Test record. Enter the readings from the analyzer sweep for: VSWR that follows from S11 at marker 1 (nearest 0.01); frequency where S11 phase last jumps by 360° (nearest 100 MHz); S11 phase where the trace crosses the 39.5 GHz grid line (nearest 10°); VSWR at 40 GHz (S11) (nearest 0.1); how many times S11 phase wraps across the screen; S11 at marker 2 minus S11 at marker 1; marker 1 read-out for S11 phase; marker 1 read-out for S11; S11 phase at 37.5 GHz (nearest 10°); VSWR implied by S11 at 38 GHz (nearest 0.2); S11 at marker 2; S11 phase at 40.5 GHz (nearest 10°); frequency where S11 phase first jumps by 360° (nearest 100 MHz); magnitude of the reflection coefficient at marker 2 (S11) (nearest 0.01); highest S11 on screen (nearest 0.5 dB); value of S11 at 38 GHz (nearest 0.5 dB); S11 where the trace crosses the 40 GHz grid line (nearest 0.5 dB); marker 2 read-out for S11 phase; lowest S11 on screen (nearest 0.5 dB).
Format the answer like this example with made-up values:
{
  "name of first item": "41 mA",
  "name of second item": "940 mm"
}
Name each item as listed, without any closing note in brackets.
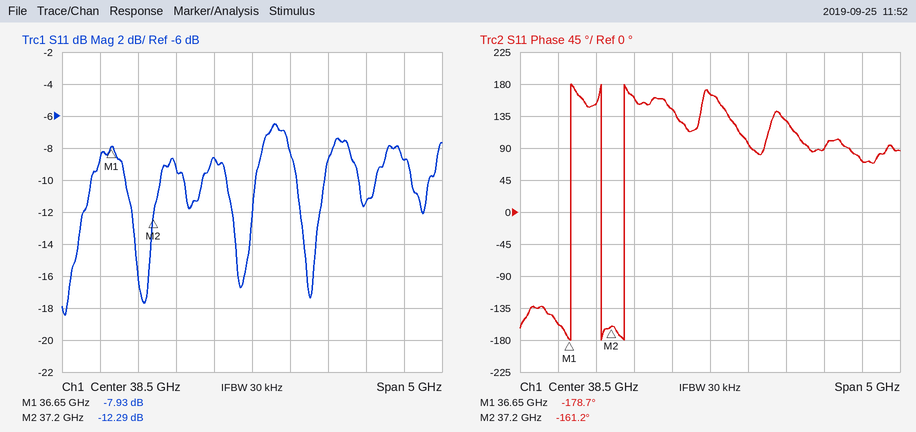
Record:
{
  "VSWR that follows from S11 at marker 1": "2.34",
  "frequency where S11 phase last jumps by 360°": "37.4 GHz",
  "S11 phase where the trace crosses the 39.5 GHz grid line": "130°",
  "VSWR at 40 GHz (S11)": "1.7",
  "how many times S11 phase wraps across the screen": "3",
  "S11 at marker 2 minus S11 at marker 1": "-4.36 dB",
  "marker 1 read-out for S11 phase": "-178.7°",
  "marker 1 read-out for S11": "-7.93 dB",
  "S11 phase at 37.5 GHz": "160°",
  "VSWR implied by S11 at 38 GHz": "2.2",
  "S11 at marker 2": "-12.29 dB",
  "S11 phase at 40.5 GHz": "70°",
  "frequency where S11 phase first jumps by 360°": "36.7 GHz",
  "magnitude of the reflection coefficient at marker 2 (S11)": "0.24",
  "highest S11 on screen": "-6.5 dB",
  "value of S11 at 38 GHz": "-8.5 dB",
  "S11 where the trace crosses the 40 GHz grid line": "-11.5 dB",
  "marker 2 read-out for S11 phase": "-161.2°",
  "lowest S11 on screen": "-18.5 dB"
}
